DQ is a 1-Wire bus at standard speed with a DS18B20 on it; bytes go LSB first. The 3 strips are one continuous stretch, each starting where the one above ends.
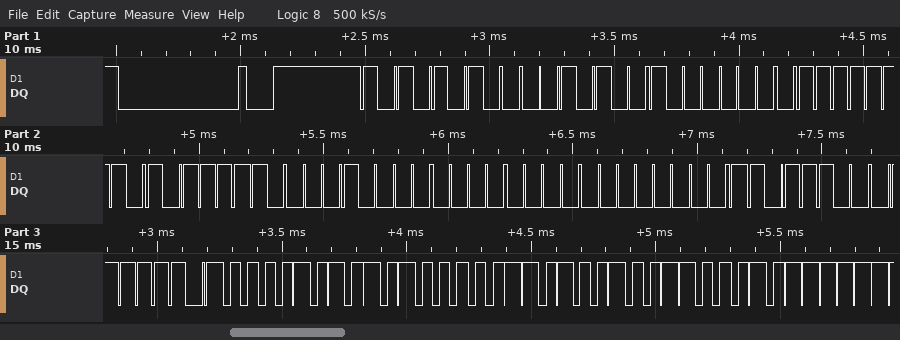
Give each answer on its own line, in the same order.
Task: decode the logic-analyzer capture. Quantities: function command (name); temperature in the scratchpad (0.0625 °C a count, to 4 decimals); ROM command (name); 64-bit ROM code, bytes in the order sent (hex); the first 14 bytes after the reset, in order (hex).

Read Scratchpad
85.0000 °C
Match ROM
28 01 7F 7D 08 00 00 3B
55 28 01 7F 7D 08 00 00 3B BE 50 05 4B 46
